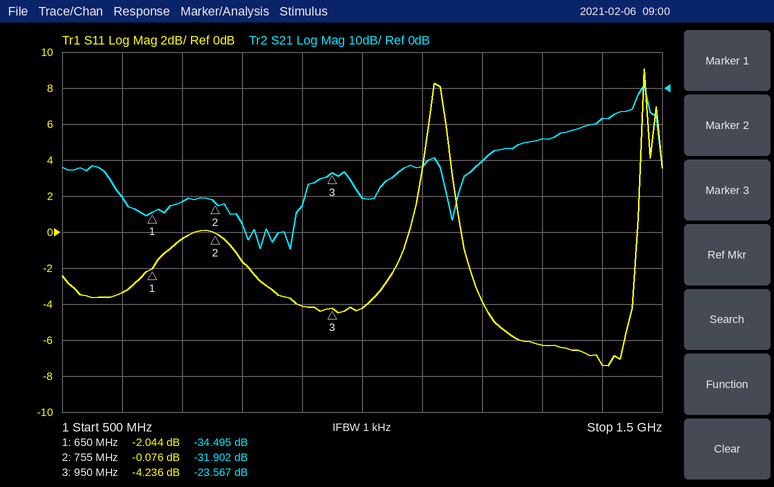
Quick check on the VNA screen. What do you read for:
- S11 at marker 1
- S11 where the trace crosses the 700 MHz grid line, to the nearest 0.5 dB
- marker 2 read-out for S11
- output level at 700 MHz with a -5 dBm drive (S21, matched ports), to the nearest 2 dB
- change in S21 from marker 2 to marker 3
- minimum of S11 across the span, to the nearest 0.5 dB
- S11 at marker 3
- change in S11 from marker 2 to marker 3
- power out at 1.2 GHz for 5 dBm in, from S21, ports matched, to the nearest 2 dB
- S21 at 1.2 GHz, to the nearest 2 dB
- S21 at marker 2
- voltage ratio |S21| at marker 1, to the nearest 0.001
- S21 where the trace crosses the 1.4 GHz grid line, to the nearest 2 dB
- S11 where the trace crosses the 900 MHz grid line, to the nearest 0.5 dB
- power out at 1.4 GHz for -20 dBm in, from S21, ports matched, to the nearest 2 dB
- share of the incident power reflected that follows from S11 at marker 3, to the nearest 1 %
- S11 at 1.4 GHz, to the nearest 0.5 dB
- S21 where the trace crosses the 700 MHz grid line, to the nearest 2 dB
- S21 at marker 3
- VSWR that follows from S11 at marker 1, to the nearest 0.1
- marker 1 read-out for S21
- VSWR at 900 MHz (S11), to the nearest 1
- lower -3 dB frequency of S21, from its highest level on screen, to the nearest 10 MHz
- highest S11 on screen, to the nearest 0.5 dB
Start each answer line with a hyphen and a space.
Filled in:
- -2.044 dB
- -0.5 dB
- -0.076 dB
- -36 dBm
- 8.335 dB
- -7.5 dB
- -4.236 dB
- -4.160 dB
- -16 dBm
- -20 dB
- -31.902 dB
- 0.019
- -8 dB
- -4.0 dB
- -28 dBm
- 38 %
- -7.5 dB
- -32 dB
- -23.567 dB
- 8.5
- -34.495 dB
- 4
- 1.46 GHz
- 9.0 dB
